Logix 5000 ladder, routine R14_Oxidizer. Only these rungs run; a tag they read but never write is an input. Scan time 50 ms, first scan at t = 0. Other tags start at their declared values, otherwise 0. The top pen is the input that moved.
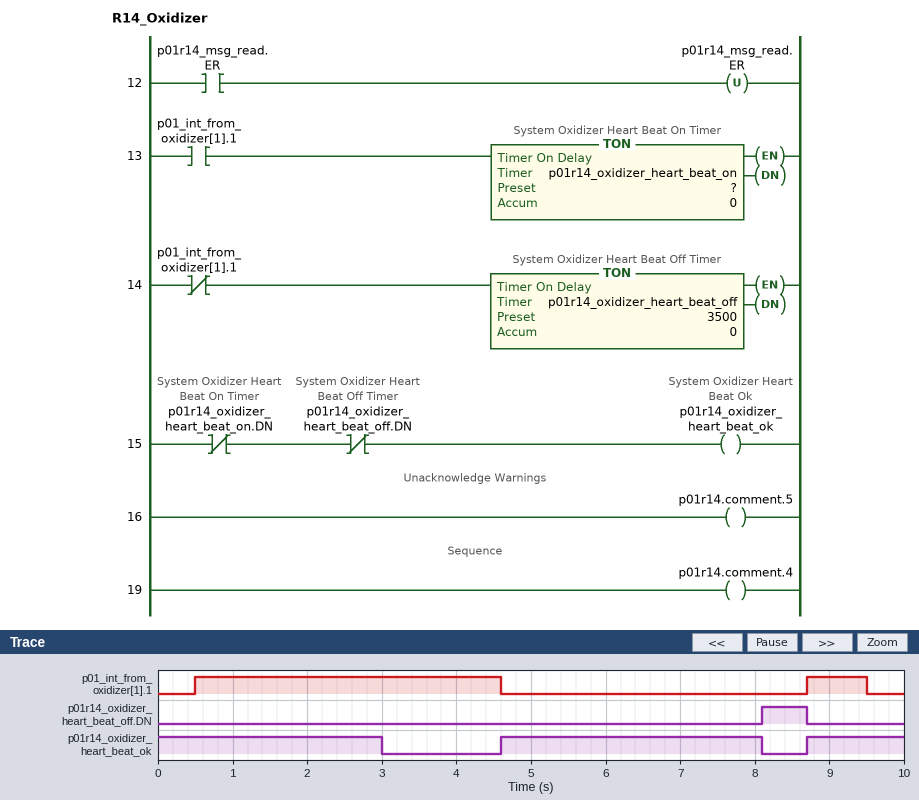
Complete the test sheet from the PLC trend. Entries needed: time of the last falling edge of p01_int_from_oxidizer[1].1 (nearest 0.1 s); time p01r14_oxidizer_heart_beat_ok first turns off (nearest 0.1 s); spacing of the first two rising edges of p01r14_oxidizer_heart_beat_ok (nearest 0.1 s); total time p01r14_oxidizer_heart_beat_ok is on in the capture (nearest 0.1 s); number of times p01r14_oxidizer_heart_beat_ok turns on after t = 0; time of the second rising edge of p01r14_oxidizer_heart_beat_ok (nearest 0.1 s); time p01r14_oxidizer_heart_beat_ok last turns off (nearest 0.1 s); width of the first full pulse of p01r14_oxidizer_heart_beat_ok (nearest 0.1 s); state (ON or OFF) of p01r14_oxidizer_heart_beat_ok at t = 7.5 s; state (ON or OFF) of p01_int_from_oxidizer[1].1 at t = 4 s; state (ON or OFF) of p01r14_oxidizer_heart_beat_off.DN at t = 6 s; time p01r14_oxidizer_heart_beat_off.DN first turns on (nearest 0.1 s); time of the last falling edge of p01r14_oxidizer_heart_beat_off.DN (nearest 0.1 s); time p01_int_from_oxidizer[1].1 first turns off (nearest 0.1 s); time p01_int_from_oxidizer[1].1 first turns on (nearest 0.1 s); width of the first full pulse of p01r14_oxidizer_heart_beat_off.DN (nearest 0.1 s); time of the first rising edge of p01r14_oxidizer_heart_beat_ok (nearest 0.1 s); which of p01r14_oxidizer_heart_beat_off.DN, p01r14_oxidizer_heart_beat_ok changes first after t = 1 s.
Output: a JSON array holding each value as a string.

["9.5 s", "3.0 s", "4.1 s", "7.8 s", "2", "8.7 s", "8.1 s", "3.5 s", "ON", "ON", "OFF", "8.1 s", "8.7 s", "4.6 s", "0.5 s", "0.6 s", "4.6 s", "p01r14_oxidizer_heart_beat_ok"]
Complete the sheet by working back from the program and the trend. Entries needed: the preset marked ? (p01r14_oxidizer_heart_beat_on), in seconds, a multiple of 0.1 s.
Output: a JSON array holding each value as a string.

["2.5 s"]
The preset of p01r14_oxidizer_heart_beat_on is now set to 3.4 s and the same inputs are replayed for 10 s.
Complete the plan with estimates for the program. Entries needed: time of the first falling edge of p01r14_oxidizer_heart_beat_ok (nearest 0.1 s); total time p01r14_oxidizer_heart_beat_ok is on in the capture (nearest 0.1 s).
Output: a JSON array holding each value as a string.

["3.9 s", "8.7 s"]
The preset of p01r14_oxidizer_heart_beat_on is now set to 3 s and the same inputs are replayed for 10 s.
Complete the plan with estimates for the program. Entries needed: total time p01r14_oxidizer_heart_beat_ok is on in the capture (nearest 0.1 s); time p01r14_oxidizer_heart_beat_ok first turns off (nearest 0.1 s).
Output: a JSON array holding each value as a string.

["8.3 s", "3.5 s"]
